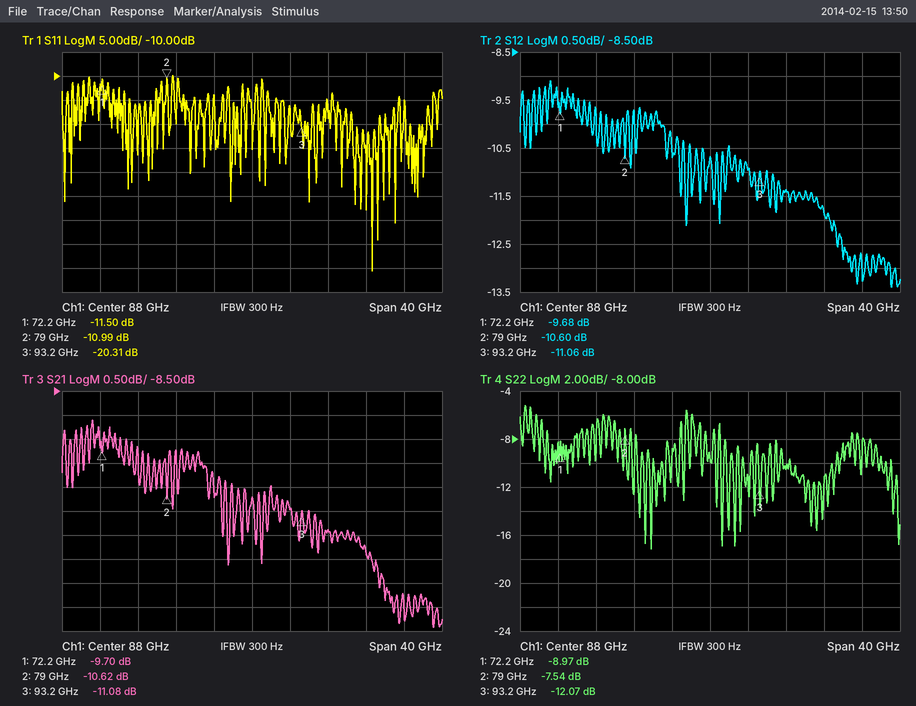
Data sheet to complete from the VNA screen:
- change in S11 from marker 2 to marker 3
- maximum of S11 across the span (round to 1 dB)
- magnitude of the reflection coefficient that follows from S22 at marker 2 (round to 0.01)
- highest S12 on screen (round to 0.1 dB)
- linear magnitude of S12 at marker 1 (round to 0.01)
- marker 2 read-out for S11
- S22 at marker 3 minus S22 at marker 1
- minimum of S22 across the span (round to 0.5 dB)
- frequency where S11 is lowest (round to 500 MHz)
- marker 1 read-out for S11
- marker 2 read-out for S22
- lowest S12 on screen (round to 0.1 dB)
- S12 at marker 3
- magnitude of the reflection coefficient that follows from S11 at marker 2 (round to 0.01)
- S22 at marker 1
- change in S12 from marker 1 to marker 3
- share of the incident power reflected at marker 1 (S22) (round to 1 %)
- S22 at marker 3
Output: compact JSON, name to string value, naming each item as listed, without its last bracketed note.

{"change in S11 from marker 2 to marker 3": "-9.32 dB", "maximum of S11 across the span": "-10 dB", "magnitude of the reflection coefficient that follows from S22 at marker 2": "0.42", "highest S12 on screen": "-9.1 dB", "linear magnitude of S12 at marker 1": "0.33", "marker 2 read-out for S11": "-10.99 dB", "S22 at marker 3 minus S22 at marker 1": "-3.10 dB", "minimum of S22 across the span": "-17.0 dB", "frequency where S11 is lowest": "100.5 GHz", "marker 1 read-out for S11": "-11.50 dB", "marker 2 read-out for S22": "-7.54 dB", "lowest S12 on screen": "-13.4 dB", "S12 at marker 3": "-11.06 dB", "magnitude of the reflection coefficient that follows from S11 at marker 2": "0.28", "S22 at marker 1": "-8.97 dB", "change in S12 from marker 1 to marker 3": "-1.38 dB", "share of the incident power reflected at marker 1 (S22)": "13 %", "S22 at marker 3": "-12.07 dB"}
